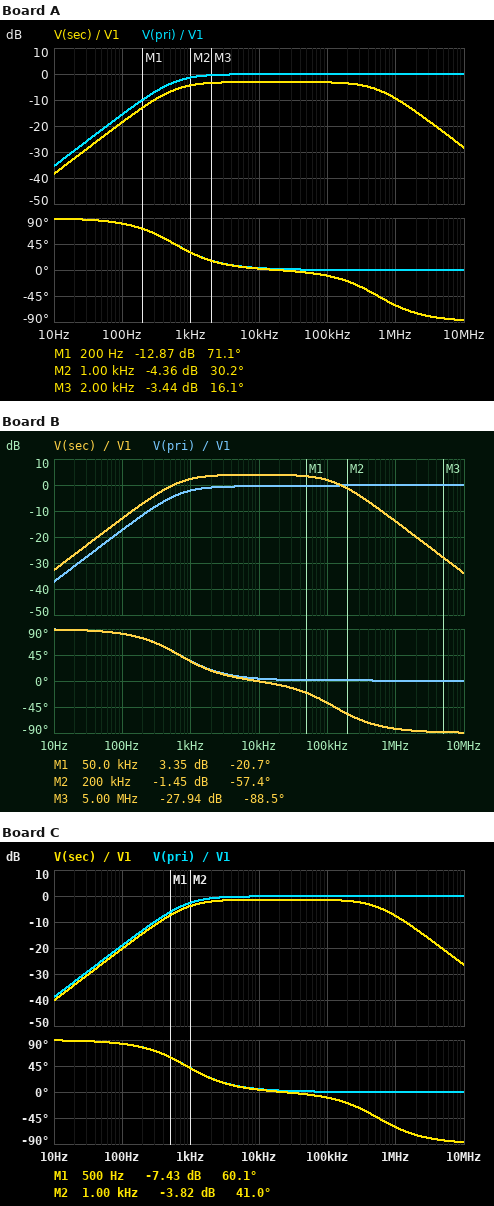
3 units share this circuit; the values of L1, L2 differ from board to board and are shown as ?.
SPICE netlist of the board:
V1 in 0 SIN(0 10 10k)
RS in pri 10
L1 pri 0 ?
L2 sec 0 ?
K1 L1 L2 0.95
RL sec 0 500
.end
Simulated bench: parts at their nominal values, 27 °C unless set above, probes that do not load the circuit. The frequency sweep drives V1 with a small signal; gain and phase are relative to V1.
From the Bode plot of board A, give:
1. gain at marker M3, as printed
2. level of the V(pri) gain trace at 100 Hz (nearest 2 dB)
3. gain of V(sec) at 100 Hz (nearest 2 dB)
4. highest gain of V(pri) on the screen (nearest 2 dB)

-3.44 dB
-16 dB
-18 dB
0 dB
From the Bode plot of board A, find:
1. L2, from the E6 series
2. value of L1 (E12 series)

1.5 mH
2.7 mH
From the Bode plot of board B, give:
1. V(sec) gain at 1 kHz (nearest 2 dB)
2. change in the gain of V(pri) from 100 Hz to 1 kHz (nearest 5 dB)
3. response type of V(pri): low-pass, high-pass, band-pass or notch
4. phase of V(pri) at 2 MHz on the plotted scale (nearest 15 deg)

2 dB
15 dB
high-pass
0 deg
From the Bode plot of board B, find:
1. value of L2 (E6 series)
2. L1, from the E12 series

6.8 mH
2.2 mH
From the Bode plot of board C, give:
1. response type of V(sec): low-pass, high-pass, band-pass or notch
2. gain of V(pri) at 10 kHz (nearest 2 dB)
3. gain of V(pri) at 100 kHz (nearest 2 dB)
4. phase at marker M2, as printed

band-pass
0 dB
0 dB
41.0 deg
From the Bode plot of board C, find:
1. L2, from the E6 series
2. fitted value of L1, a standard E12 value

1.5 mH
1.8 mH
